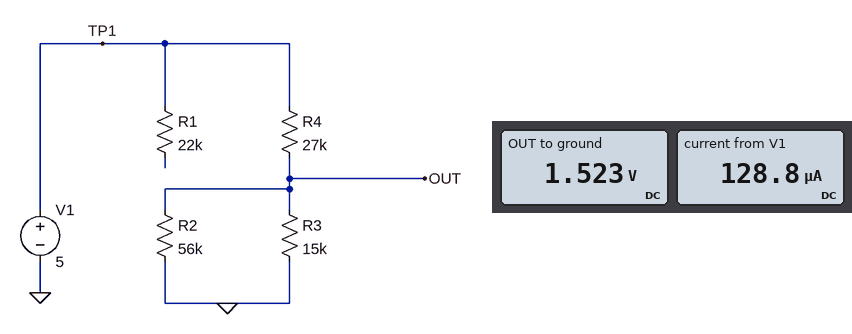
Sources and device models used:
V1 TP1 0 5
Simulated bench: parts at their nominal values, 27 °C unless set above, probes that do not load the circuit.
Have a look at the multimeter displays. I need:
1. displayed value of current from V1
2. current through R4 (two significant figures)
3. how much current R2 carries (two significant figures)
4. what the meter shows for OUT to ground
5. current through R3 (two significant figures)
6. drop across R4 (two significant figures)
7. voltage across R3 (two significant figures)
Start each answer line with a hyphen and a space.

- 128.8 µA
- 130 µA
- 27 µA
- 1.523 V
- 100 µA
- 3.5 V
- 1.5 V
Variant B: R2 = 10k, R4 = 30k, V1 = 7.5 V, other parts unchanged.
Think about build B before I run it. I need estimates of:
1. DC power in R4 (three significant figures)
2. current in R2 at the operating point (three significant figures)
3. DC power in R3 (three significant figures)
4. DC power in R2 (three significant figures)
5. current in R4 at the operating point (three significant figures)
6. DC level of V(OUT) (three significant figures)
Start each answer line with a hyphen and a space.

- 1.30 mW
- 125 µA
- 104 µW
- 156 µW
- 208 µA
- 1.25 V
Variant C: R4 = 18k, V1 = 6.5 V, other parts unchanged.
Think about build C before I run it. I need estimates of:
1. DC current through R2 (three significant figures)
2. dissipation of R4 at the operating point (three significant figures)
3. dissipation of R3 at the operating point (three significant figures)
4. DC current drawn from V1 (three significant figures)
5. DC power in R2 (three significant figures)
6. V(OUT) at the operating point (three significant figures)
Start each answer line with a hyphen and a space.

- 46.0 µA
- 855 µW
- 443 µW
- 218 µA
- 119 µW
- 2.58 V
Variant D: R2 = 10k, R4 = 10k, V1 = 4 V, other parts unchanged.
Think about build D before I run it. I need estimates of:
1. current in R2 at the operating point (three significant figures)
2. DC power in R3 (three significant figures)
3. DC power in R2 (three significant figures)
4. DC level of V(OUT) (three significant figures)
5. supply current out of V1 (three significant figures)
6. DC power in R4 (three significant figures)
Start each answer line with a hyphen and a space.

- 150 µA
- 150 µW
- 225 µW
- 1.50 V
- 250 µA
- 625 µW
